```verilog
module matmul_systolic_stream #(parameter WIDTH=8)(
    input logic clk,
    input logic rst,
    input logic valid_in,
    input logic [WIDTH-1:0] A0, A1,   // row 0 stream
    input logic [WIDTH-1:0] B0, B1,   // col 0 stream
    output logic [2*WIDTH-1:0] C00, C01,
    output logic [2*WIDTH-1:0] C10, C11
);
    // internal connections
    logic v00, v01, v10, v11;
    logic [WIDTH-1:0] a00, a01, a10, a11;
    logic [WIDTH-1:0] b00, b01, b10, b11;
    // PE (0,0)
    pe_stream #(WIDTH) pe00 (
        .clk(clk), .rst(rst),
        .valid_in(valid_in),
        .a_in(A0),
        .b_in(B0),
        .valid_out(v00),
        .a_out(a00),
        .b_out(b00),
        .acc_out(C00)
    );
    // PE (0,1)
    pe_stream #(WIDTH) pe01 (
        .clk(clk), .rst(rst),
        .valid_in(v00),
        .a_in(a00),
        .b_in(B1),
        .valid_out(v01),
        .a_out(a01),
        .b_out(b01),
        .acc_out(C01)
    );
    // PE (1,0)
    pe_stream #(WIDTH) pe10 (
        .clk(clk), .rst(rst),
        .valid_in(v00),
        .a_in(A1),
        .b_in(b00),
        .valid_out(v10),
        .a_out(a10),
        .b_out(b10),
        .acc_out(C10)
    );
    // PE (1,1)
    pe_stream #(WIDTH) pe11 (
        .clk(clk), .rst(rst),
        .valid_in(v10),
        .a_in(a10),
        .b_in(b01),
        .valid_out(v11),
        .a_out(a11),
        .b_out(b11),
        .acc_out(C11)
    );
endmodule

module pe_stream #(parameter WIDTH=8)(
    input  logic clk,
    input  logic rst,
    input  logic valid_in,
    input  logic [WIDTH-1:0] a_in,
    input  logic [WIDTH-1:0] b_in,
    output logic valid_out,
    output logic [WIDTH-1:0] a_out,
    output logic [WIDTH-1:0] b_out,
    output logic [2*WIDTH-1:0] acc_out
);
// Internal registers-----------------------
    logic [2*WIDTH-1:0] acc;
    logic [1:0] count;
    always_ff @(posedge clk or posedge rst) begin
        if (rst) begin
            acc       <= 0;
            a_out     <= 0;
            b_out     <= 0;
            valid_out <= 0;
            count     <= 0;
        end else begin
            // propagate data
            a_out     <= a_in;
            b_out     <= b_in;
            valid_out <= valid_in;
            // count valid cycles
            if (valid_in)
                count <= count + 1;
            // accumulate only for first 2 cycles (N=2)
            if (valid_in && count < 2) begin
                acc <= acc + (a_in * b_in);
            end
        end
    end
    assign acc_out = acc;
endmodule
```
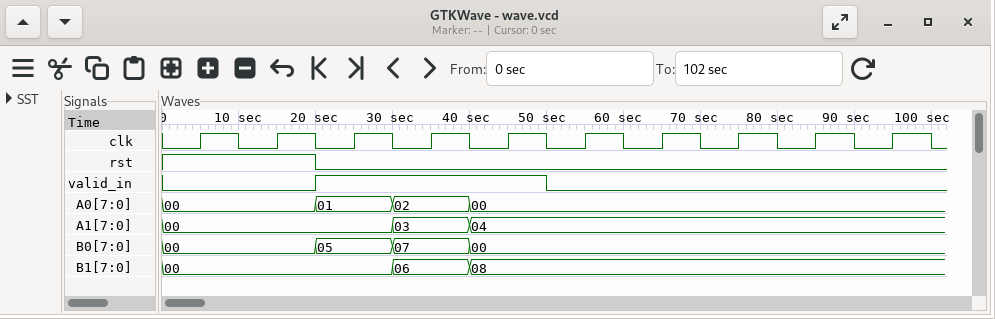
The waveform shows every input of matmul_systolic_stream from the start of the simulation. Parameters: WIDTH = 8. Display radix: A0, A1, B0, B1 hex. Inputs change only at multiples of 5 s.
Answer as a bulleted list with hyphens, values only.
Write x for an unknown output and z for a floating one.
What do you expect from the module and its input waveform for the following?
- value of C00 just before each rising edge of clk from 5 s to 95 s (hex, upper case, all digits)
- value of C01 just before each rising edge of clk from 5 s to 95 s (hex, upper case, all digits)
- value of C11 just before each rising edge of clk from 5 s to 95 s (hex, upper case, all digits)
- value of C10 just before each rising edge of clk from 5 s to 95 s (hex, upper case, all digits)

- 0000, 0000, 0000, 0005, 0013, 0013, 0013, 0013, 0013, 0013
- 0000, 0000, 0000, 0000, 0006, 0016, 0016, 0016, 0016, 0016
- 0000, 0000, 0000, 0000, 0000, 0012, 0032, 0032, 0032, 0032
- 0000, 0000, 0000, 0000, 000F, 002B, 002B, 002B, 002B, 002B
